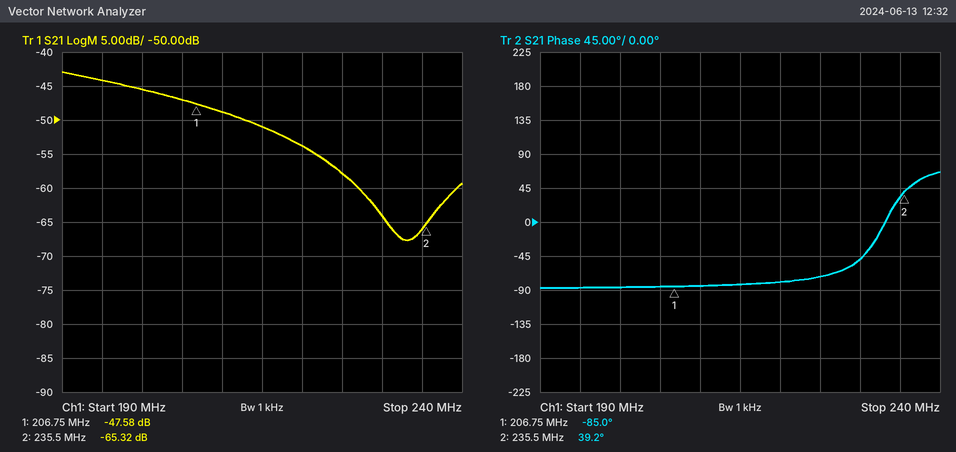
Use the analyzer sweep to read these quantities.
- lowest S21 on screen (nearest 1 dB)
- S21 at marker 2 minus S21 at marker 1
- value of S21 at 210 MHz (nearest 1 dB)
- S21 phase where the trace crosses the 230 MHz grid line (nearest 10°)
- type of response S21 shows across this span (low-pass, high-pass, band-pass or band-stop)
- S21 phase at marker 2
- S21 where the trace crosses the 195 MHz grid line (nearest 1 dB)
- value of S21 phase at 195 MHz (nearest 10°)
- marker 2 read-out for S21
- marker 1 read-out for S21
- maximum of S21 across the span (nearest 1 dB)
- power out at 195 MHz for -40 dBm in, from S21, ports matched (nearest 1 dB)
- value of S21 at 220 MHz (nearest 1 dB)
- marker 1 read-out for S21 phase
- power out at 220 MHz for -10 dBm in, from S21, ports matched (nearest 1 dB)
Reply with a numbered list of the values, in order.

1. -68 dB
2. -17.74 dB
3. -49 dB
4. -50°
5. low-pass
6. 39.2°
7. -44 dB
8. -90°
9. -65.32 dB
10. -47.58 dB
11. -43 dB
12. -84 dBm
13. -54 dB
14. -85.0°
15. -64 dBm
